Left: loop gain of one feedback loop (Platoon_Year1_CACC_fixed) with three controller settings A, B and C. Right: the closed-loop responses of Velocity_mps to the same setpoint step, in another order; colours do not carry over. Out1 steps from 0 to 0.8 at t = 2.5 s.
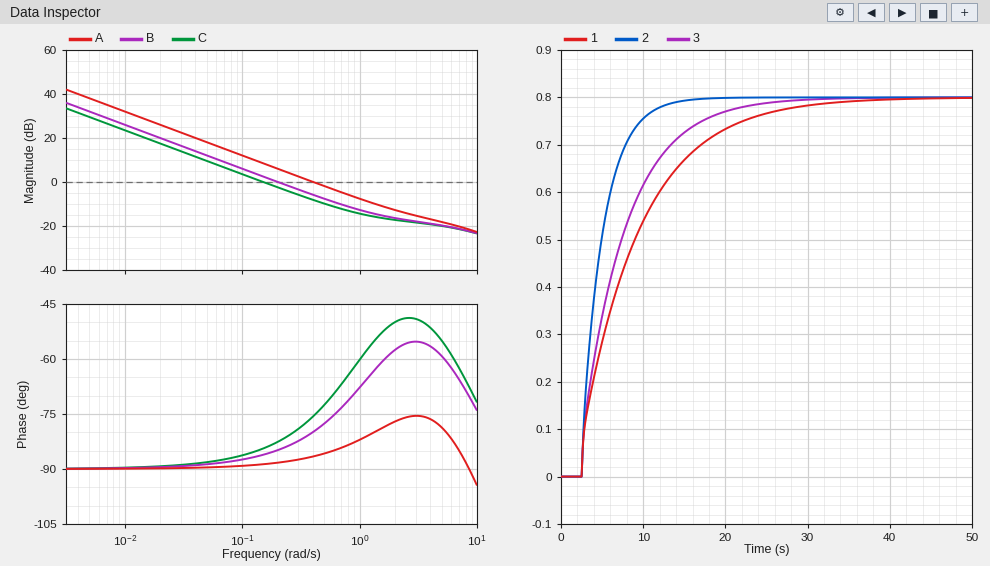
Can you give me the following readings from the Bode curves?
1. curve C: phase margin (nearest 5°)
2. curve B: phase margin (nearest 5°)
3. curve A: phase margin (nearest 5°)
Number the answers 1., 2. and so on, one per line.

1. 95°
2. 95°
3. 95°
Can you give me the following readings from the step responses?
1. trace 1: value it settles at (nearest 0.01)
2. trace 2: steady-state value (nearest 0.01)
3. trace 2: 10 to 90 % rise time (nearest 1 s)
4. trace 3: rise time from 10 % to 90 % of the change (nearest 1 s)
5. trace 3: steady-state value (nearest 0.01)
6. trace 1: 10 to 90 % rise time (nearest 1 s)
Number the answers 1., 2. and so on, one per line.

1. 0.80
2. 0.80
3. 6 s
4. 12 s
5. 0.80
6. 16 s
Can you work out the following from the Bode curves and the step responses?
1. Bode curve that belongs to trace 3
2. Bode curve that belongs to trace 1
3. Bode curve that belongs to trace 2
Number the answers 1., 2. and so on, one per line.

1. B
2. C
3. A
